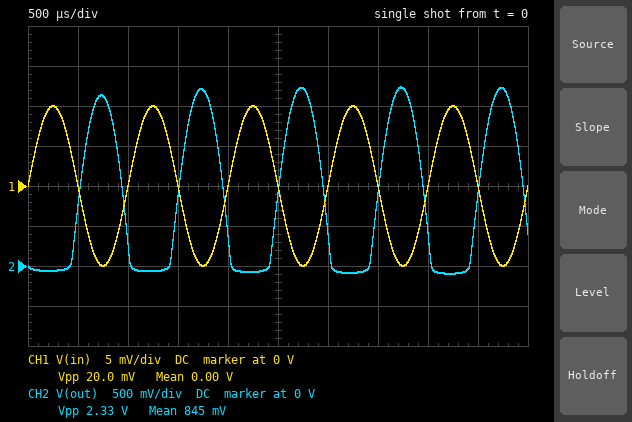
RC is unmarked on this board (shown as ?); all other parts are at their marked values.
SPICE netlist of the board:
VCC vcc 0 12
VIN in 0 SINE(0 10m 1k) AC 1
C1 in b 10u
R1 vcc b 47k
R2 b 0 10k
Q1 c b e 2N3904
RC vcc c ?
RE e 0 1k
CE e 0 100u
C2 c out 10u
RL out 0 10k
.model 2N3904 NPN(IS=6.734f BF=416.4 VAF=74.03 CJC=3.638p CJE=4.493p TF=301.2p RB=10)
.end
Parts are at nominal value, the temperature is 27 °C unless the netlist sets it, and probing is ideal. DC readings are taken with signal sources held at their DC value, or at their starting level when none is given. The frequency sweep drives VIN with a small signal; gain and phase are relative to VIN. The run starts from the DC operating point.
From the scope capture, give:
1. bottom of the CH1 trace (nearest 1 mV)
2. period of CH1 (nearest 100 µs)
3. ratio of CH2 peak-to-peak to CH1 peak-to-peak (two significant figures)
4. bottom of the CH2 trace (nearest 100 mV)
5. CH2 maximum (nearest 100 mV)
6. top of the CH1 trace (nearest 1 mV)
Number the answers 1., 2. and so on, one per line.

1. -10 mV
2. 1.0 ms
3. 120
4. -100 mV
5. 2.2 V
6. 10 mV
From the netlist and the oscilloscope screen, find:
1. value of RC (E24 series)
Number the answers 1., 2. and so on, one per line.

1. 8.2 kΩ
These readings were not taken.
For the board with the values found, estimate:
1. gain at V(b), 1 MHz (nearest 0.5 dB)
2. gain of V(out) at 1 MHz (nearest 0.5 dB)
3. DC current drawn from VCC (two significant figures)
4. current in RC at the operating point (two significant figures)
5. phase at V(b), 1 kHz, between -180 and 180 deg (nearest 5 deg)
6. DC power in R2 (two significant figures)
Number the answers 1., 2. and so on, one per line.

1. 0 dB
2. 31.0 dB
3. 1.5 mA
4. 1.3 mA
5. 15 deg
6. 390 µW
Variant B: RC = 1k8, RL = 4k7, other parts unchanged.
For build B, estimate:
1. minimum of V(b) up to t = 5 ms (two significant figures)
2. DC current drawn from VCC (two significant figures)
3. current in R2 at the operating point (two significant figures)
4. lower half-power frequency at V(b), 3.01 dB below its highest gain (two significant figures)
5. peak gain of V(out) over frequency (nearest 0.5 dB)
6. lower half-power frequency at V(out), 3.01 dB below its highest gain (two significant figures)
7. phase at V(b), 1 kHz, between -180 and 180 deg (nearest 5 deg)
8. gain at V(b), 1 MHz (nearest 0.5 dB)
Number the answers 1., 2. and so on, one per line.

1. 2.1 V
2. 1.6 mA
3. 210 µA
4. 2.0 Hz
5. 37.0 dB
6. 88 Hz
7. 0 deg
8. 0 dB
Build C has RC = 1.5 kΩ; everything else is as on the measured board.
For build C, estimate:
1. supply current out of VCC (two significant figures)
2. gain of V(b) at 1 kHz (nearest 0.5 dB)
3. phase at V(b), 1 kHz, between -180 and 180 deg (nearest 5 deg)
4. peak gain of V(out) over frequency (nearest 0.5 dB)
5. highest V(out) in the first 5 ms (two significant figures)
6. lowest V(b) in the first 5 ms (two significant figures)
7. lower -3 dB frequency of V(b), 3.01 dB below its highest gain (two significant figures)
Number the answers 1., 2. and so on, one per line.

1. 1.6 mA
2. 0 dB
3. 0 deg
4. 37.0 dB
5. 620 mV
6. 2.1 V
7. 2.0 Hz
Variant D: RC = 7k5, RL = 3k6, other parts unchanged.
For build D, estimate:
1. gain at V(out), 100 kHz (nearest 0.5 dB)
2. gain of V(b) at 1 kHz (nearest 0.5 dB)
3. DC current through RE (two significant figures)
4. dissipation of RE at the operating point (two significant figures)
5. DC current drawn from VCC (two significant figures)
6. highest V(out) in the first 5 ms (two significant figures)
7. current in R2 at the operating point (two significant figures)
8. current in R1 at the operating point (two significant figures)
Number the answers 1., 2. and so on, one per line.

1. 40.0 dB
2. 0 dB
3. 1.4 mA
4. 1.9 mW
5. 1.6 mA
6. 1.4 V
7. 210 µA
8. 210 µA
